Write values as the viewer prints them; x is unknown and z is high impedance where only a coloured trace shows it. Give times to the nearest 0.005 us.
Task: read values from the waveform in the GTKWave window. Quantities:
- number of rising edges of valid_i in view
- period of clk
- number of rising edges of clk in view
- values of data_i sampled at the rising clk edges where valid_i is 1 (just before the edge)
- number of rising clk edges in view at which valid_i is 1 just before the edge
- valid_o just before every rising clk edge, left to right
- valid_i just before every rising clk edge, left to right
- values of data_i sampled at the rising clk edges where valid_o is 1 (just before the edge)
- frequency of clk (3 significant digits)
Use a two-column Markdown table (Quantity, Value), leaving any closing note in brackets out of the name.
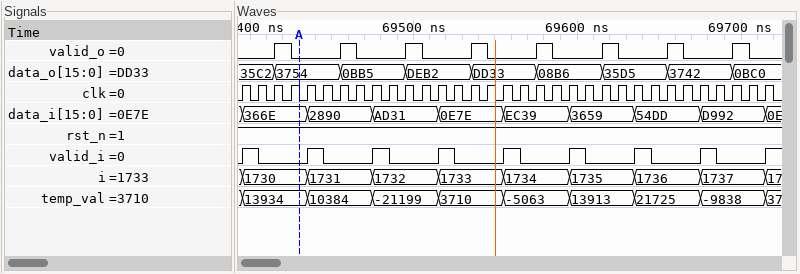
| Quantity | Value |
|---|---|
| number of rising edges of valid_i in view | 9 |
| period of clk | 0.01 us |
| number of rising edges of clk in view | 33 |
| values of data_i sampled at the rising clk edges where valid_i is 1 | 366E, 2890, AD31, 0E7E, EC39, 3659, 54DD, D992 |
| number of rising clk edges in view at which valid_i is 1 just before the edge | 8 |
| valid_o just before every rising clk edge, left to right | 0 0 0 1 0 0 0 1 0 0 0 1 0 0 0 1 0 0 0 1 0 0 0 1 0 0 0 1 0 0 0 1 0 |
| valid_i just before every rising clk edge, left to right | 0 1 0 0 0 1 0 0 0 1 0 0 0 1 0 0 0 1 0 0 0 1 0 0 0 1 0 0 0 1 0 0 0 |
| values of data_i sampled at the rising clk edges where valid_o is 1 | 366E, 2890, AD31, 0E7E, EC39, 3659, 54DD, D992 |
| frequency of clk | 100 MHz |
